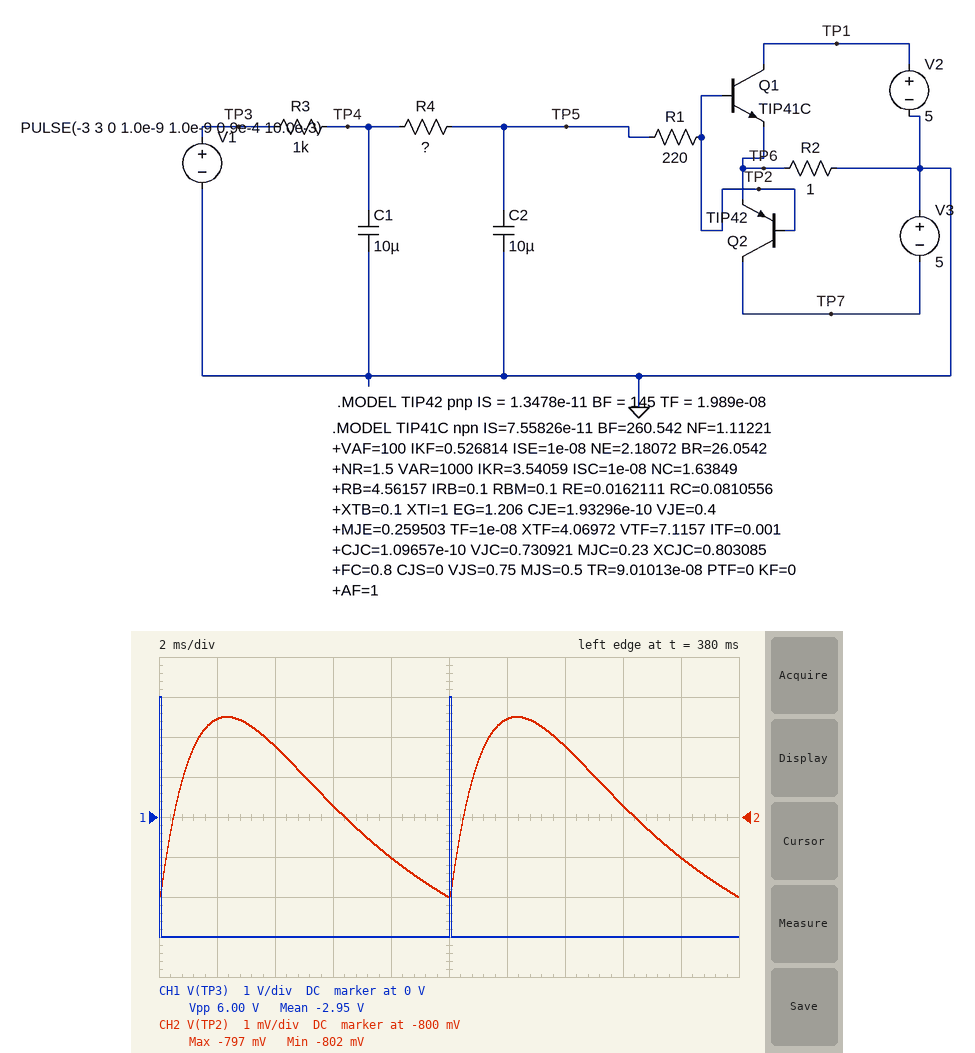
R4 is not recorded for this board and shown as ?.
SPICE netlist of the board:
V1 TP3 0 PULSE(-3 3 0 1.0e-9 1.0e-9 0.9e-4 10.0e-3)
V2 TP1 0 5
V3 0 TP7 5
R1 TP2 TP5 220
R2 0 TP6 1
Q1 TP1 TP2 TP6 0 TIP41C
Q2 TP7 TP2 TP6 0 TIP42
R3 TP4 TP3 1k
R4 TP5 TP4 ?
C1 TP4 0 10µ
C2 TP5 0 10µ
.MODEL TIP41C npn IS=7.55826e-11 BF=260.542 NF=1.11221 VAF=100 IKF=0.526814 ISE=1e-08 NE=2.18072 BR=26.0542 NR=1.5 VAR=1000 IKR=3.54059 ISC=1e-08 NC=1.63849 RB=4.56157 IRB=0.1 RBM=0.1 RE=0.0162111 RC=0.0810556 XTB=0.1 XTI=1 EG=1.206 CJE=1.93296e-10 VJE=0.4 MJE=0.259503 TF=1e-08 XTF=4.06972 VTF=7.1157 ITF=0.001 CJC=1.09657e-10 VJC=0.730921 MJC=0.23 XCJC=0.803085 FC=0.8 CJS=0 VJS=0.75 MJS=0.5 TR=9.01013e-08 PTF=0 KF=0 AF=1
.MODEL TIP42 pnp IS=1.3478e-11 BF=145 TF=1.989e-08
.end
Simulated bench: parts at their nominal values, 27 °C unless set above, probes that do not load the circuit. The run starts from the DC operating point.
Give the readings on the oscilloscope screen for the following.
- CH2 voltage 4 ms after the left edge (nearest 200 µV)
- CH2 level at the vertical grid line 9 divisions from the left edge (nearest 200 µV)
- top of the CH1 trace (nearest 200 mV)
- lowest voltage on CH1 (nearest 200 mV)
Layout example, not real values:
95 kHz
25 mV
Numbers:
-798.2 mV
-801.0 mV
3.0 V
-3.0 V
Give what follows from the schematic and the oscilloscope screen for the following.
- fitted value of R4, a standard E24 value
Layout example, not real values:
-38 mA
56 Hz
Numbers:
390 Ω
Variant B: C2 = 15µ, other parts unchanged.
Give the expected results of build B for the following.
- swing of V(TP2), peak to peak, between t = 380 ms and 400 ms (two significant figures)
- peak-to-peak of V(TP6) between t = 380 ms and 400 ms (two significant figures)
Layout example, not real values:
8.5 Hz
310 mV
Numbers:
3.4 mV
3.0 mV
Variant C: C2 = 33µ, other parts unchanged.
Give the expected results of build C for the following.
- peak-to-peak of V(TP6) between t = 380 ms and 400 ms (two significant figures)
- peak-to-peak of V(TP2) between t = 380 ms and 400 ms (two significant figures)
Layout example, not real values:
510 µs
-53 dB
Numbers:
1.6 mV
1.8 mV
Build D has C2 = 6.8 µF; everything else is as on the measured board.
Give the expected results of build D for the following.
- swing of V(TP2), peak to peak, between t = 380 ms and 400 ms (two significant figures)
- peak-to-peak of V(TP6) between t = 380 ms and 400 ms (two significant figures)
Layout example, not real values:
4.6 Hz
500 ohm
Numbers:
5.6 mV
4.9 mV
